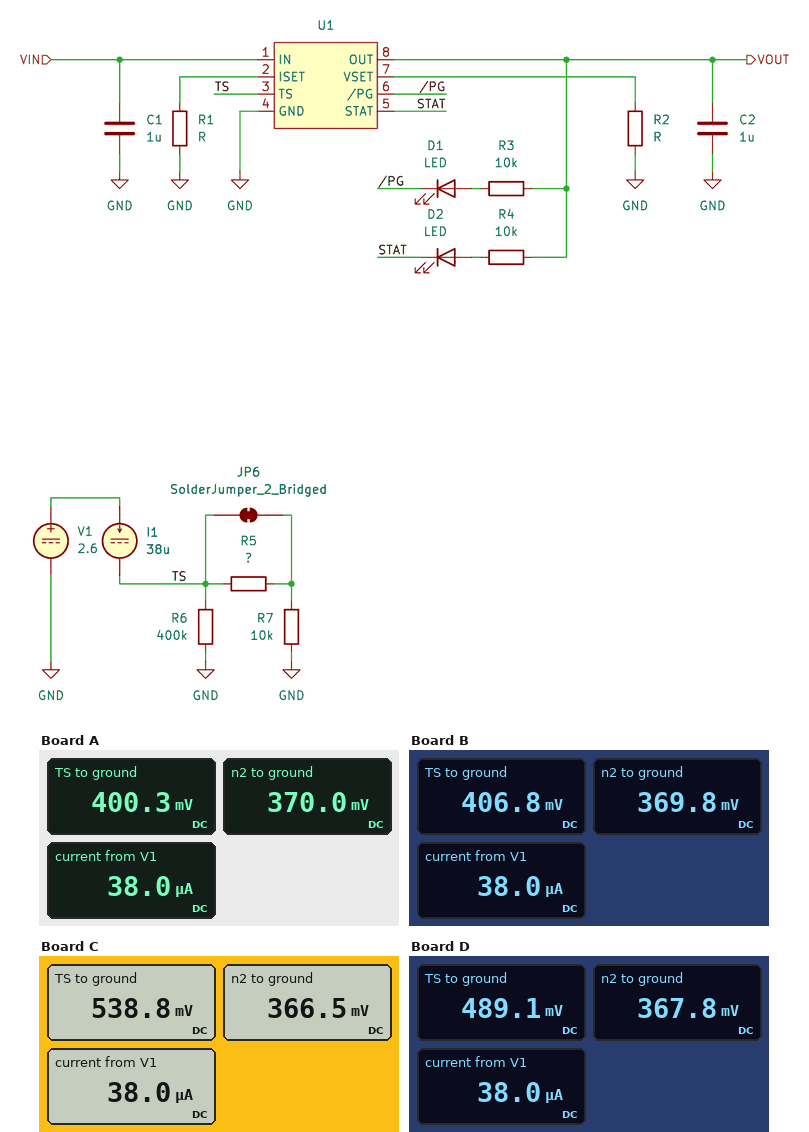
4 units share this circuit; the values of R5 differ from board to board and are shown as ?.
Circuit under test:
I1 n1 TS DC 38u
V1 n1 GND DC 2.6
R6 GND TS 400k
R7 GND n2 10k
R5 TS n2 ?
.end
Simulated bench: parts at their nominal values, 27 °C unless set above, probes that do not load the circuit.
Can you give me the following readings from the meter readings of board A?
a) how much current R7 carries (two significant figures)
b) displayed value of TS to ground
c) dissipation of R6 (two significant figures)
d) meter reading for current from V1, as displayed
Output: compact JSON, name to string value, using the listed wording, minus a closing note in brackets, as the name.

{"how much current R7 carries": "37 µA", "displayed value of TS to ground": "400.3 mV", "dissipation of R6": "400 nW", "meter reading for current from V1, as displayed": "38.0 µA"}
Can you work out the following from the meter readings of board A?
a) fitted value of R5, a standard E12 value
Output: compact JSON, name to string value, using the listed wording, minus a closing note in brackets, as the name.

{"fitted value of R5, a standard E12 value": "820 Ω"}
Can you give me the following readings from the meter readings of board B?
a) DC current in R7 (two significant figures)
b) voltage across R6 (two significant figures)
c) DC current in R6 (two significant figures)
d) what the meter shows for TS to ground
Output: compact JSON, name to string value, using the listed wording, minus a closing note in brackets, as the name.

{"DC current in R7": "37 µA", "voltage across R6": "410 mV", "DC current in R6": "1.0 µA", "what the meter shows for TS to ground": "406.8 mV"}
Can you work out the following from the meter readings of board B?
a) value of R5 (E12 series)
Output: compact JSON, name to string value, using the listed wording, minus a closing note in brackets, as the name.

{"value of R5": "1 kΩ"}
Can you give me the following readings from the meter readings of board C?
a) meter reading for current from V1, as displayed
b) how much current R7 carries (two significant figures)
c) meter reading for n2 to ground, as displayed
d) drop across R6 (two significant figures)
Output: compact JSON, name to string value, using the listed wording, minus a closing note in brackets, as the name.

{"meter reading for current from V1, as displayed": "38.0 µA", "how much current R7 carries": "37 µA", "meter reading for n2 to ground, as displayed": "366.5 mV", "drop across R6": "540 mV"}
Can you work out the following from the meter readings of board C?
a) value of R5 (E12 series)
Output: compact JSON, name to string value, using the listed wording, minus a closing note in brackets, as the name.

{"value of R5": "4.7 kΩ"}
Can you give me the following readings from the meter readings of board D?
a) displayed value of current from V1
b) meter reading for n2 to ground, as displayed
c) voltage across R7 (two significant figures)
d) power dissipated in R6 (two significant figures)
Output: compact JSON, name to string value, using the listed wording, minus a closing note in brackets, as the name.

{"displayed value of current from V1": "38.0 µA", "meter reading for n2 to ground, as displayed": "367.8 mV", "voltage across R7": "370 mV", "power dissipated in R6": "600 nW"}
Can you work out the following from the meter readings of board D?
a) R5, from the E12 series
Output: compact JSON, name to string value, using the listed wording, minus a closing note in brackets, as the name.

{"R5, from the E12 series": "3.3 kΩ"}
